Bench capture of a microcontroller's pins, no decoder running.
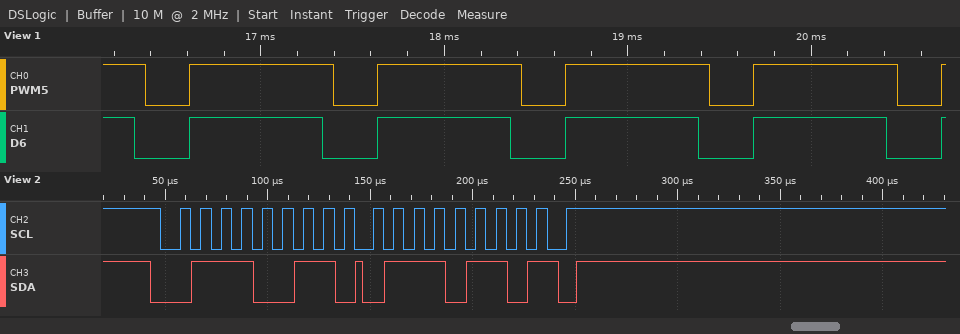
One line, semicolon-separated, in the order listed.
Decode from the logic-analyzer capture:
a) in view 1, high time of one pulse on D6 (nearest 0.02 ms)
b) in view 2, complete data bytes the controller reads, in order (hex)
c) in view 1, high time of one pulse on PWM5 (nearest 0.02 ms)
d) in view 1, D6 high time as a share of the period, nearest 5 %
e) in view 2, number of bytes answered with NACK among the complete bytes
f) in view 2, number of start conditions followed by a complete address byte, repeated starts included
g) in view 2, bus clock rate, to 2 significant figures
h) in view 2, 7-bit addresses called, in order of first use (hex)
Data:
0.72 ms; 76; 0.78 ms; 70 %; 1; 1; 100 kHz; 0x39
